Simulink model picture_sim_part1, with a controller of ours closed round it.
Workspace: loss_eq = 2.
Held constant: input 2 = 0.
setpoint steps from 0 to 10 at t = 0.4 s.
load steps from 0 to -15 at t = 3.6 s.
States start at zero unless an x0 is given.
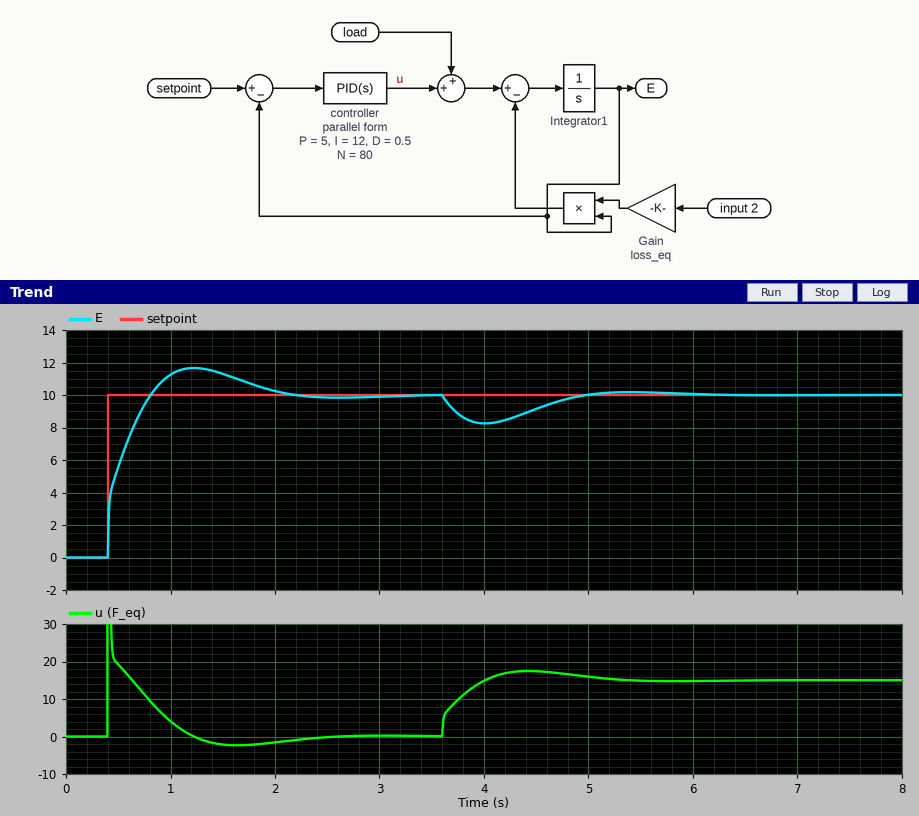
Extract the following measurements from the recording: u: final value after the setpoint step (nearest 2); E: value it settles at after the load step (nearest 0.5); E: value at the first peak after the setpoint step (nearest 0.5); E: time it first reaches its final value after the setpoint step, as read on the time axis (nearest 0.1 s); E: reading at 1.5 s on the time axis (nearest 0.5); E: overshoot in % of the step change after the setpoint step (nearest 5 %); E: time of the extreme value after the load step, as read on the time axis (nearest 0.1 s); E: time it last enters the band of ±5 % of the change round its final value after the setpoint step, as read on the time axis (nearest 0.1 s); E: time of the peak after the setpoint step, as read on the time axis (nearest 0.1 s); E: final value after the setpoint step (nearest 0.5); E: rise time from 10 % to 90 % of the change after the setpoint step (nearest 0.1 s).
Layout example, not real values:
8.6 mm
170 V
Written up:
0
10.0
11.5
0.8 s
11.5
15 %
4.0 s
1.9 s
1.2 s
10.0
0.3 s
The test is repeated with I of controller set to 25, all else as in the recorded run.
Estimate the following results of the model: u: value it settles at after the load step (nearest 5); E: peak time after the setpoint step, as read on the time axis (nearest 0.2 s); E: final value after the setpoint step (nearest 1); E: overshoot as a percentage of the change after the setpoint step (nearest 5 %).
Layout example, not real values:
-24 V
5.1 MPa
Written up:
15
1.0 s
10
25 %
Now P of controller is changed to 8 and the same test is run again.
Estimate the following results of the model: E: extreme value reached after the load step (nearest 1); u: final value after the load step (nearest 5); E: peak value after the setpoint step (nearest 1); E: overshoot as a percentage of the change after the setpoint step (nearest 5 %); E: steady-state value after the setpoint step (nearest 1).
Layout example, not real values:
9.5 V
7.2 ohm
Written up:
9
15
11
10 %
10
